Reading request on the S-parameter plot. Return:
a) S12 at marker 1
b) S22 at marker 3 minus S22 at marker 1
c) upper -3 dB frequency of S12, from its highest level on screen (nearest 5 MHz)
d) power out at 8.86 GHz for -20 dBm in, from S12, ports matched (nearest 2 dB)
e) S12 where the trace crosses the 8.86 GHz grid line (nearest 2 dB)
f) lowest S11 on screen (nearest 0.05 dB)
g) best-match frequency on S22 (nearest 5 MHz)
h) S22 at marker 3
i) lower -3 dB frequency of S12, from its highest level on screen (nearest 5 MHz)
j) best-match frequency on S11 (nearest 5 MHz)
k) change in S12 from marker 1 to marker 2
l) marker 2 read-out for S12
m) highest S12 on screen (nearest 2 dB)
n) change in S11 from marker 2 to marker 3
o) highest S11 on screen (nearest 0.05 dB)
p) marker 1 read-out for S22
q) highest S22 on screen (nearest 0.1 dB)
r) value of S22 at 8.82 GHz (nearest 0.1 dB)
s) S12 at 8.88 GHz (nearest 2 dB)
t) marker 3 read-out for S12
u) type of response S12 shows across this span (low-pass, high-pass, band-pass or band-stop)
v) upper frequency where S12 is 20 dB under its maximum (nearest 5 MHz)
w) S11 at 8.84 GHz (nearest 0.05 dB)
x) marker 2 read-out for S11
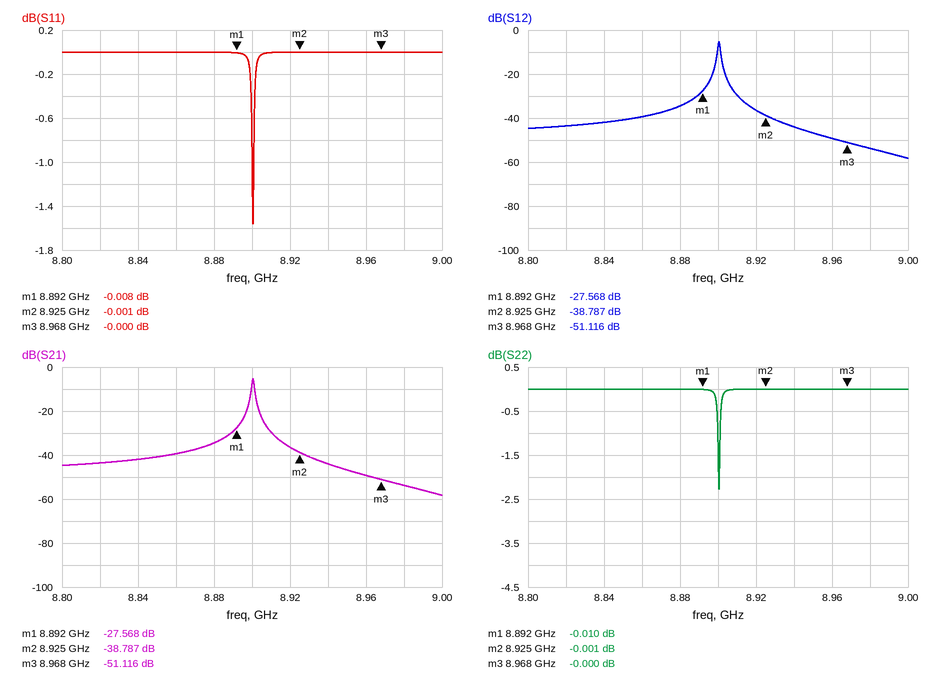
-27.568 dB
0.010 dB
8.900 GHz
-60 dBm
-40 dB
-1.55 dB
8.900 GHz
-0.000 dB
8.900 GHz
8.900 GHz
-11.219 dB
-38.787 dB
-6 dB
0.001 dB
0.00 dB
-0.010 dB
0.0 dB
0.0 dB
-34 dB
-51.116 dB
band-pass
8.905 GHz
0.00 dB
-0.001 dB
